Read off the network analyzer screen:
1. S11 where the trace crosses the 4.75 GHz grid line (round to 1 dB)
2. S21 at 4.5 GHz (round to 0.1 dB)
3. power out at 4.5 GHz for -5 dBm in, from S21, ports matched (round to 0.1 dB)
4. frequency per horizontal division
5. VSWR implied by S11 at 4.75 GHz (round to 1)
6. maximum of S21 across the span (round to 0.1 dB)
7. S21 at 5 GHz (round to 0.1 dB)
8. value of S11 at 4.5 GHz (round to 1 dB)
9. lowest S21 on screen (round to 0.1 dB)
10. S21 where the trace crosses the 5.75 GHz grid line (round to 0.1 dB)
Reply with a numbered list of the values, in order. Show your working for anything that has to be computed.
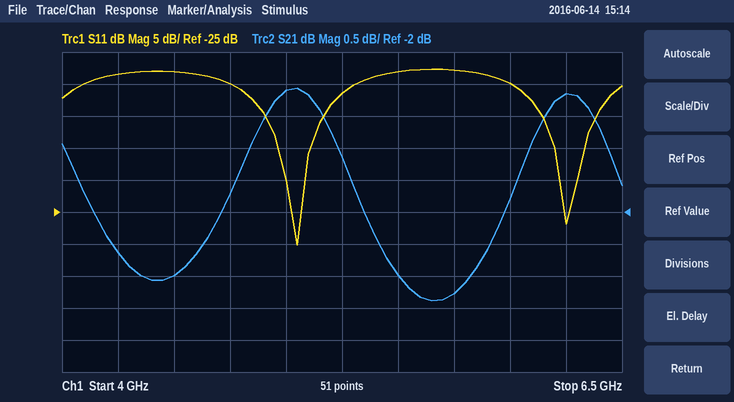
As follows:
1. -5 dB
2. -3.0 dB
3. -5 dBm + (-3.0 dB) = -8.0 dBm
4. 250 MHz
5. |Γ| = 10^(-5/20) = 0.5623; VSWR = (1 + 0.5623)/(1 − 0.5623) ≈ 4
6. -0.1 dB
7. -0.1 dB
8. -3 dB
9. -3.4 dB
10. -3.3 dB
